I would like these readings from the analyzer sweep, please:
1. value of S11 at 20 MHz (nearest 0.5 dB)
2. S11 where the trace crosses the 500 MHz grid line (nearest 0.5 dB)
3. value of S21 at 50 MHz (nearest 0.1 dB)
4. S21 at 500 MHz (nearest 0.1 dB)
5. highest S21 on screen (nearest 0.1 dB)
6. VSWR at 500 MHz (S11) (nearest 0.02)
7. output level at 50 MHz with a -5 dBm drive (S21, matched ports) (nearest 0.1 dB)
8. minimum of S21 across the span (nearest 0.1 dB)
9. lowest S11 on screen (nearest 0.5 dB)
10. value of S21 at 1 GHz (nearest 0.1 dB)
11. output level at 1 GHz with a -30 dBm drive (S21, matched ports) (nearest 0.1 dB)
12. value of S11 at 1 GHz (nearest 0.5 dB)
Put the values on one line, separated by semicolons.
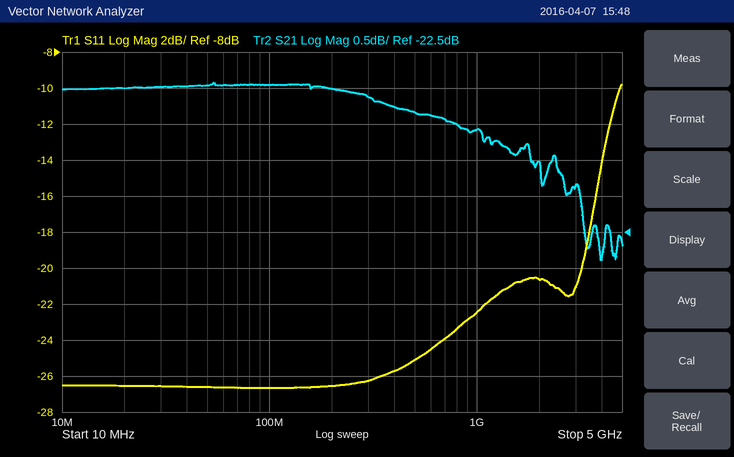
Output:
-26.5 dB; -25.0 dB; -20.5 dB; -20.8 dB; -20.4 dB; 1.12; -25.5 dBm; -22.9 dB; -26.5 dB; -21.1 dB; -51.1 dBm; -22.5 dB
